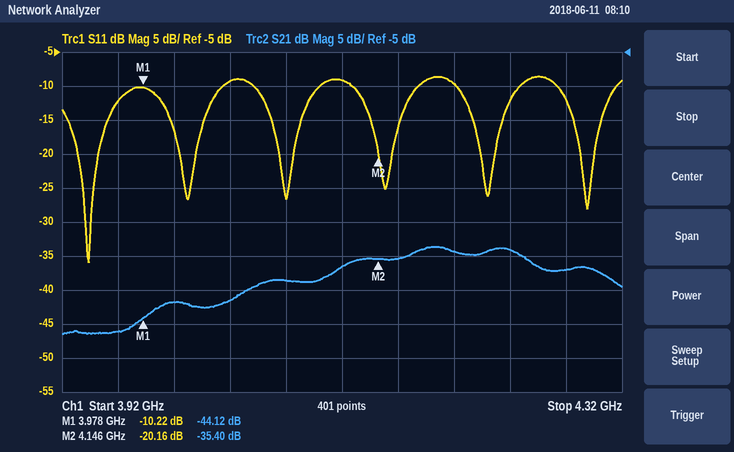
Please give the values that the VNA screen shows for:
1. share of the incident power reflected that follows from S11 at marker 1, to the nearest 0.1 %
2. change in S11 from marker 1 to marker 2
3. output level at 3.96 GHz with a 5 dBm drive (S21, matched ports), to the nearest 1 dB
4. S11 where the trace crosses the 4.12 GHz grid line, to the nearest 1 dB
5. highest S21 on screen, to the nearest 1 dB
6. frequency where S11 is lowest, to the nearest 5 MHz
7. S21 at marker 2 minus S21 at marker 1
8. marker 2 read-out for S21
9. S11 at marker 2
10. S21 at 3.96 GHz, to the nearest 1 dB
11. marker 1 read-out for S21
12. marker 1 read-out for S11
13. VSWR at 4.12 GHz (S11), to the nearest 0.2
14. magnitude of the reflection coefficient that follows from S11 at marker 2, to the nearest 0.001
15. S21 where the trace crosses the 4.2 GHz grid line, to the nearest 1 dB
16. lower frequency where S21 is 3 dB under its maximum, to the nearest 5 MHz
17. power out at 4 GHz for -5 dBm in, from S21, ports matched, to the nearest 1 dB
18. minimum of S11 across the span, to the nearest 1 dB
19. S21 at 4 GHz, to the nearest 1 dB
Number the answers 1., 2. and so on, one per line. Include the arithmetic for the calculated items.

1. 10^(-10.22/10) ≈ 9.5 %
2. -20.16 − (-10.22) = -9.94 dB
3. 5 dBm + (-46 dB) = -41 dBm
4. -9 dB
5. -34 dB
6. 3.940 GHz
7. -35.4 − (-44.12) = 8.72 dB
8. -35.40 dB
9. -20.16 dB
10. -46 dB
11. -44.12 dB
12. -10.22 dB
13. |Γ| = 10^(-9/20) = 0.3548; VSWR = (1 + 0.3548)/(1 − 0.3548) ≈ 2.10, so 2.0 to the nearest 0.2
14. 10^(-20.16/20) ≈ 0.098
15. -34 dB
16. 4.120 GHz
17. -5 dBm + (-42 dB) = -47 dBm
18. -36 dB
19. -42 dB
